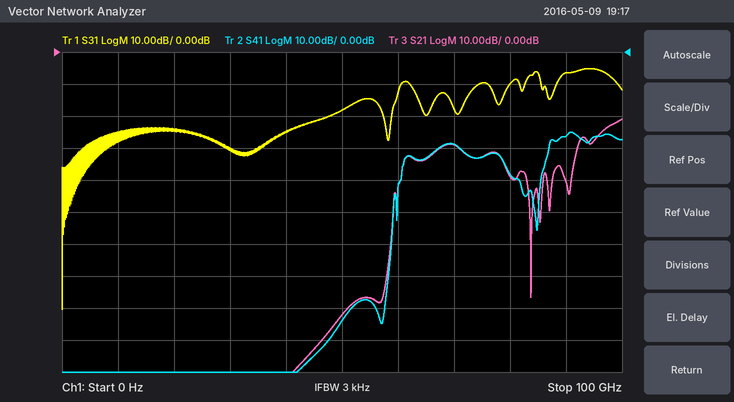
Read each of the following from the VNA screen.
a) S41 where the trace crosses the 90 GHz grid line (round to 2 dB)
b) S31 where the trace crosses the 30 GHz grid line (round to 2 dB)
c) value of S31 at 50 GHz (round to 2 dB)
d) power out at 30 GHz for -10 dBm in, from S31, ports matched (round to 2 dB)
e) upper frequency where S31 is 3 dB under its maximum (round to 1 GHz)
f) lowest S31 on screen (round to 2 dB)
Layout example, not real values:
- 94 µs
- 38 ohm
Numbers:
- -26 dB
- -30 dB
- -18 dB
- -40 dBm
- 98 GHz
- -80 dB
